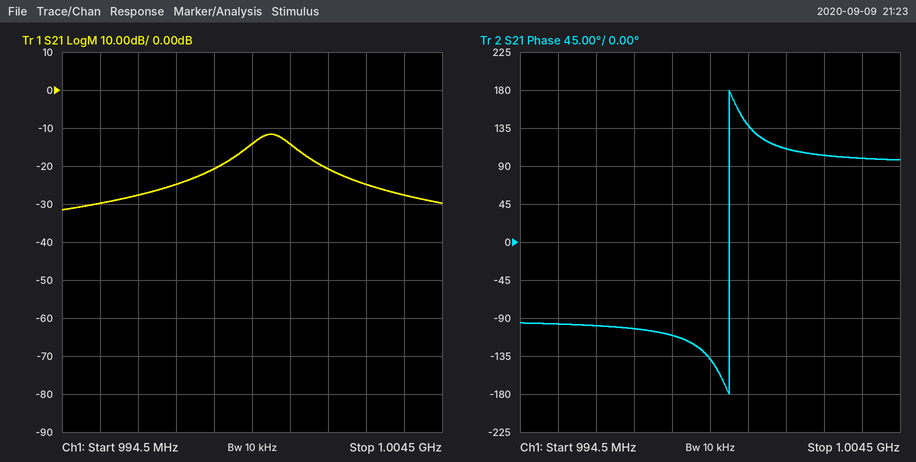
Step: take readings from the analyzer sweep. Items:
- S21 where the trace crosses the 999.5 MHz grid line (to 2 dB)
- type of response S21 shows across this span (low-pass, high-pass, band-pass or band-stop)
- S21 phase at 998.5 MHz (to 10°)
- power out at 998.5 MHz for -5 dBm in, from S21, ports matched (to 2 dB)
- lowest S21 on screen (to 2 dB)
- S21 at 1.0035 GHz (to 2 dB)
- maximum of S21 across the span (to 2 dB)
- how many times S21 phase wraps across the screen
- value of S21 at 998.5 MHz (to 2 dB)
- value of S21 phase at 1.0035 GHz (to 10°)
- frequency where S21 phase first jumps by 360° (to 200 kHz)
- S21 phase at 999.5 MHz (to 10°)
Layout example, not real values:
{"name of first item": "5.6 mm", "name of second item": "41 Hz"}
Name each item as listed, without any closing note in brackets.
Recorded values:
{"S21 where the trace crosses the 999.5 MHz grid line": "-14 dB", "type of response S21 shows across this span": "band-pass", "S21 phase at 998.5 MHz": "-110°", "power out at 998.5 MHz for -5 dBm in, from S21, ports matched": "-26 dBm", "lowest S21 on screen": "-32 dB", "S21 at 1.0035 GHz": "-28 dB", "maximum of S21 across the span": "-12 dB", "how many times S21 phase wraps across the screen": "1", "value of S21 at 998.5 MHz": "-20 dB", "value of S21 phase at 1.0035 GHz": "100°", "frequency where S21 phase first jumps by 360°": "1.0000 GHz", "S21 phase at 999.5 MHz": "-140°"}
